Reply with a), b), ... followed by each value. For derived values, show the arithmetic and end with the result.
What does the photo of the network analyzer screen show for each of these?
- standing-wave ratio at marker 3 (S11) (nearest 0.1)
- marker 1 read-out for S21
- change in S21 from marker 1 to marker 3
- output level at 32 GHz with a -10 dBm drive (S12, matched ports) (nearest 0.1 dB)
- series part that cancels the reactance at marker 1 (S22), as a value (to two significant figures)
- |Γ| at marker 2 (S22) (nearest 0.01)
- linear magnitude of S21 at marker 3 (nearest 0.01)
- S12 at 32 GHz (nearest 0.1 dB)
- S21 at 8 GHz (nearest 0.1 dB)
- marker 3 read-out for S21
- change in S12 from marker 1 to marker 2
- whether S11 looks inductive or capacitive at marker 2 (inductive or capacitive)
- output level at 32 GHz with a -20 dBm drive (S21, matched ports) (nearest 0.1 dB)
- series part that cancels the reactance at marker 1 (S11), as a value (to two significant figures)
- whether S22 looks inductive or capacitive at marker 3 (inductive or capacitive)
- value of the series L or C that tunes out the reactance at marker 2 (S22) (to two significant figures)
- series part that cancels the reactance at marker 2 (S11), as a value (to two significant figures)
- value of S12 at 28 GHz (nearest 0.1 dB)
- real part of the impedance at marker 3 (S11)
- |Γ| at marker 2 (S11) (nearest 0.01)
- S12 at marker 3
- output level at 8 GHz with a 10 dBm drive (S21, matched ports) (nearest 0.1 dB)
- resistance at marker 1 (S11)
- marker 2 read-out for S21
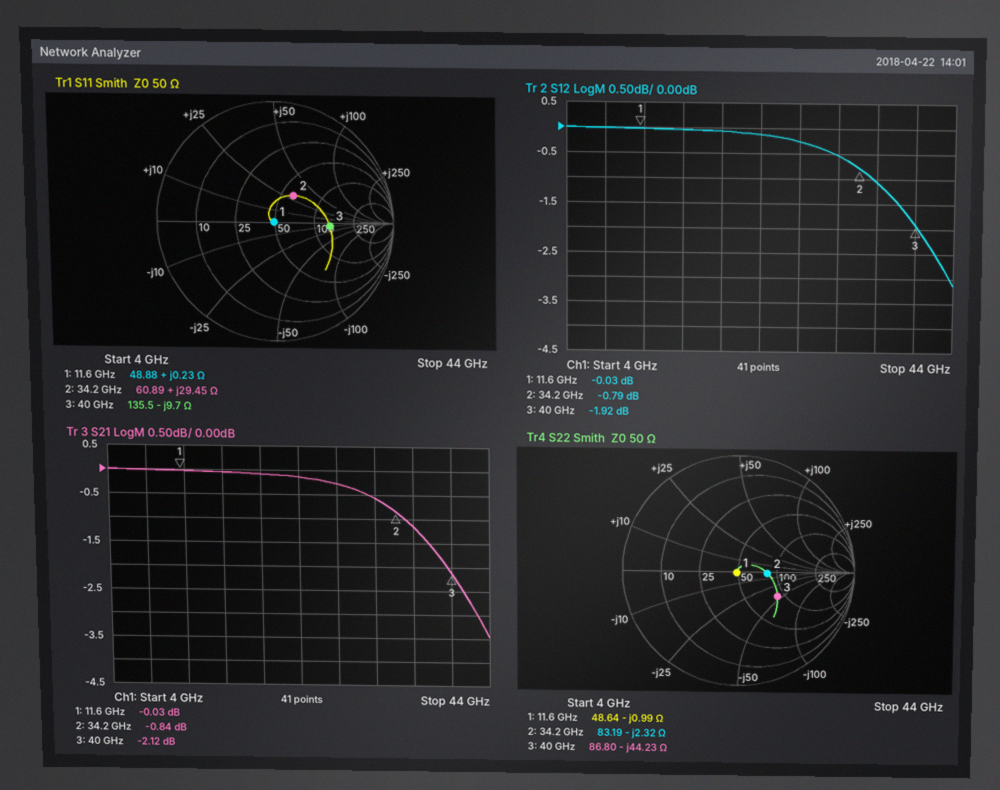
a) 2.7
b) -0.03 dB
c) -2.12 − (-0.03) = -2.09 dB
d) -10 dBm + (-0.5 dB) = -10.5 dBm
e) L = 0.99 Ω/(2π × 11.6 GHz) ≈ 14 pH
f) 0.25
g) 10^(-2.12/20) ≈ 0.78
h) -0.5 dB
i) 0.0 dB
j) -2.12 dB
k) -0.79 − (-0.03) = -0.76 dB
l) inductive
m) -20 dBm + (-0.6 dB) = -20.6 dBm
n) C = 1/(2π × 11.6 GHz × 0.23 Ω) ≈ 60 pF
o) capacitive
p) L = 2.32 Ω/(2π × 34.2 GHz) ≈ 11 pH
q) C = 1/(2π × 34.2 GHz × 29.45 Ω) ≈ 158 fF, so 160 fF to two significant figures
r) -0.3 dB
s) 135.5 Ω
t) 0.27
u) -1.92 dB
v) 10 dBm + (0.0 dB) = 10.0 dBm
w) 48.88 Ω
x) -0.84 dB
